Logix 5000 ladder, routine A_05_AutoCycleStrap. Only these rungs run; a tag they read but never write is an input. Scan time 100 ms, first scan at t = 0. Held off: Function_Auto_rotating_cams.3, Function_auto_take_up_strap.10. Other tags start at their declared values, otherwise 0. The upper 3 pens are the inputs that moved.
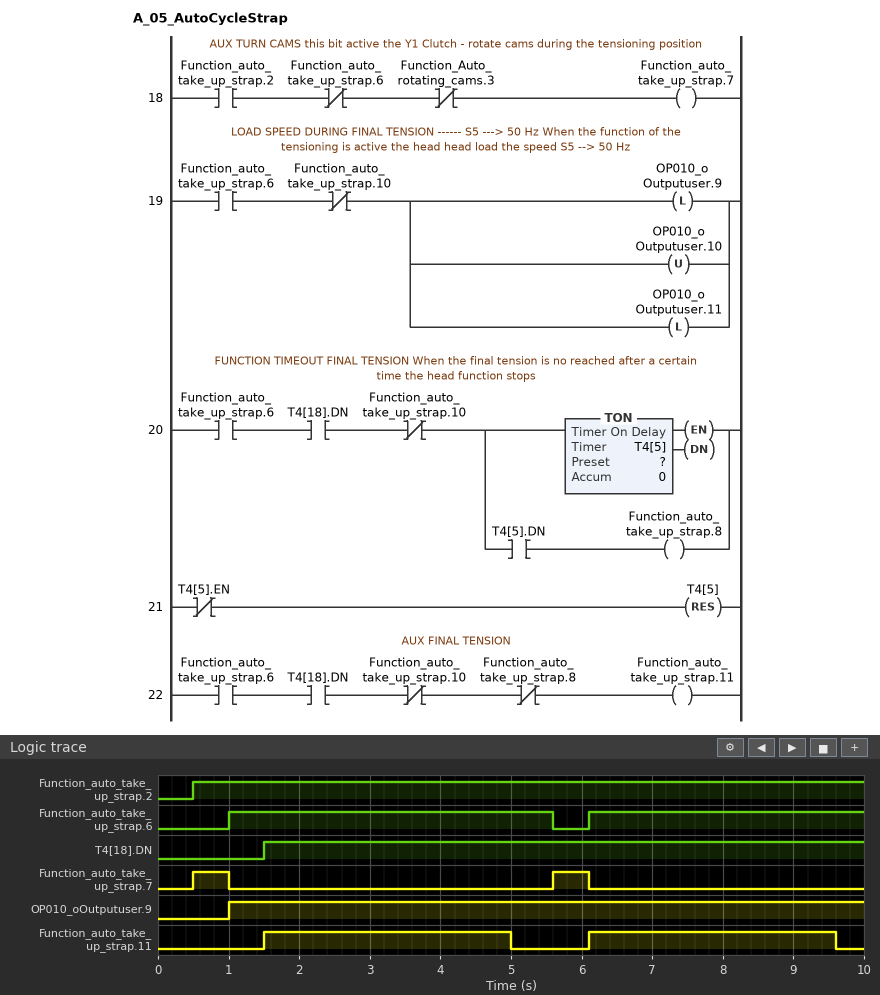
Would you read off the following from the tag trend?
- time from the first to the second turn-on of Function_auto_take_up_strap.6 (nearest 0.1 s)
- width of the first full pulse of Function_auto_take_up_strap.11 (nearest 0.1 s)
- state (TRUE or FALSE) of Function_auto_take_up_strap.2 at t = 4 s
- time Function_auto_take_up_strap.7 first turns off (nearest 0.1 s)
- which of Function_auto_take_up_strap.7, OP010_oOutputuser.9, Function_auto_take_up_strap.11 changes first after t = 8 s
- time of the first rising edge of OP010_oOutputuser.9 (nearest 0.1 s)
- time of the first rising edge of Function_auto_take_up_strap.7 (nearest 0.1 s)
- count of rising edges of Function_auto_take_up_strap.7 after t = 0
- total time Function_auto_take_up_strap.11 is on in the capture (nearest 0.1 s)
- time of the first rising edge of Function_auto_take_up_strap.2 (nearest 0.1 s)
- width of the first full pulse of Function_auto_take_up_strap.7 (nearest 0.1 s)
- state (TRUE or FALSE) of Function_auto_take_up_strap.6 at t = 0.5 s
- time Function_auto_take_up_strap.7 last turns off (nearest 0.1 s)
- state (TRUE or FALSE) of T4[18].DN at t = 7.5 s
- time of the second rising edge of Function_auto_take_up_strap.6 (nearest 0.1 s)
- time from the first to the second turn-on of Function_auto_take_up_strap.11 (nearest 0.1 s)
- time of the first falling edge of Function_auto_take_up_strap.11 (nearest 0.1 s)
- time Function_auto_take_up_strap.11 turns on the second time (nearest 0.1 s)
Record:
5.1 s
3.5 s
TRUE
1.0 s
Function_auto_take_up_strap.11
1.0 s
0.5 s
2
7.0 s
0.5 s
0.5 s
FALSE
6.1 s
TRUE
6.1 s
4.6 s
5.0 s
6.1 s
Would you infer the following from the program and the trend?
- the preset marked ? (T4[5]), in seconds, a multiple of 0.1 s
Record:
3.5 s
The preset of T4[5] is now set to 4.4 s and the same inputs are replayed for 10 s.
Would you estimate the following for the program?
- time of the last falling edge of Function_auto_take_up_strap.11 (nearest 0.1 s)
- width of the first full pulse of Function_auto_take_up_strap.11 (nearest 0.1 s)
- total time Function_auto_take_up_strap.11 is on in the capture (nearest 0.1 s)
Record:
5.6 s
4.1 s
8.0 s
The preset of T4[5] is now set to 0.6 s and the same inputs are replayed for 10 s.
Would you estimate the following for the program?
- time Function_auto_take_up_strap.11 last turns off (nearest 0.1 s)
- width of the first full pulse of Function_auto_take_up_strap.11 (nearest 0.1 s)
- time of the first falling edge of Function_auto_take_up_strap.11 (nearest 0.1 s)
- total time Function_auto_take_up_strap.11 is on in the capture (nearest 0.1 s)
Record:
6.7 s
0.6 s
2.1 s
1.2 s
